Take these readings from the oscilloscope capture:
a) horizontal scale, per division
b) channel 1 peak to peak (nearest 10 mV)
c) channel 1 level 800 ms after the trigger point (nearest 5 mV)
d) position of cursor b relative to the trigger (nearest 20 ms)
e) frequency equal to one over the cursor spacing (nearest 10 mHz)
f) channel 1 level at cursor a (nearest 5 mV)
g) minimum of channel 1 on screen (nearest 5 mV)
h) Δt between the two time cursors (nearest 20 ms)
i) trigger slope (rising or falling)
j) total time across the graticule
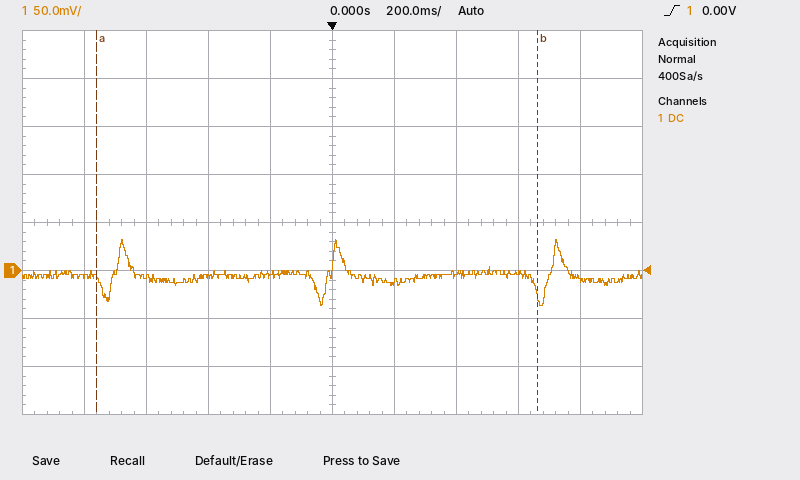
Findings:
200 ms
70 mV
-10 mV
+660 ms
700 mHz
-10 mV
-35 mV
1.42 s
rising
2 s
